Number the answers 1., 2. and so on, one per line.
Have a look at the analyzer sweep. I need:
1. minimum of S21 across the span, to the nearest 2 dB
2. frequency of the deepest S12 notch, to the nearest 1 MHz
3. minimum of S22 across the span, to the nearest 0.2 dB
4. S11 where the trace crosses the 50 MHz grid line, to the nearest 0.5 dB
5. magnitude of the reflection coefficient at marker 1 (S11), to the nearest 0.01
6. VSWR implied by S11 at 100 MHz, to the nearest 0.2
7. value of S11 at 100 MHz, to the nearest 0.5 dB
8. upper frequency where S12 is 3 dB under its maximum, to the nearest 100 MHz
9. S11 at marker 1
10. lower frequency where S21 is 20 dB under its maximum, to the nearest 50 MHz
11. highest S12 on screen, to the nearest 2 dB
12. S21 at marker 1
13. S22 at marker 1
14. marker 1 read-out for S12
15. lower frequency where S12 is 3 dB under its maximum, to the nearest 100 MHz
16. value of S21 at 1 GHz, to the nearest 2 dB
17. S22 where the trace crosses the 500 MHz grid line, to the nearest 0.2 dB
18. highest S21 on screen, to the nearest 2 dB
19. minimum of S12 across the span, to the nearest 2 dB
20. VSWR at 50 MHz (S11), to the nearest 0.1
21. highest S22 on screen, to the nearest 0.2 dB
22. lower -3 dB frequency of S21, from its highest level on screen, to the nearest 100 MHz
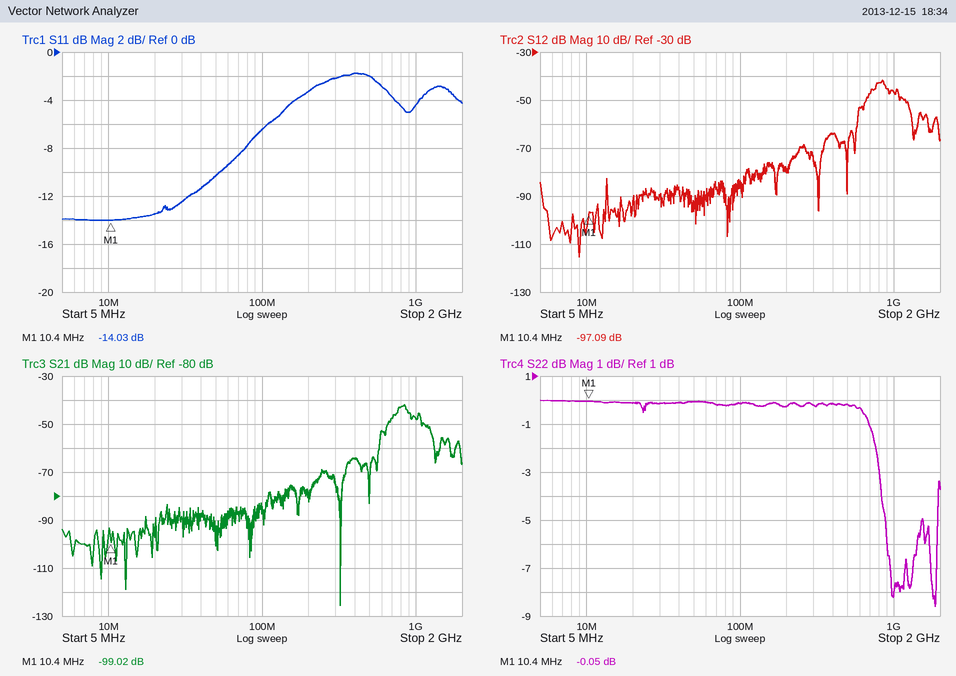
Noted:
1. -126 dB
2. 9 MHz
3. -8.6 dB
4. -10.5 dB
5. 0.20
6. 2.8
7. -6.5 dB
8. 900 MHz
9. -14.03 dB
10. 550 MHz
11. -42 dB
12. -99.02 dB
13. -0.05 dB
14. -97.09 dB
15. 800 MHz
16. -48 dB
17. -0.2 dB
18. -42 dB
19. -116 dB
20. 1.9
21. 0.0 dB
22. 800 MHz
